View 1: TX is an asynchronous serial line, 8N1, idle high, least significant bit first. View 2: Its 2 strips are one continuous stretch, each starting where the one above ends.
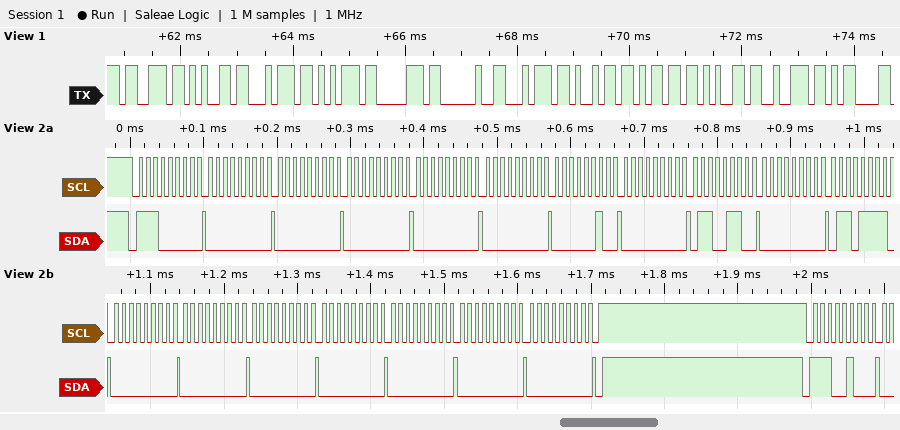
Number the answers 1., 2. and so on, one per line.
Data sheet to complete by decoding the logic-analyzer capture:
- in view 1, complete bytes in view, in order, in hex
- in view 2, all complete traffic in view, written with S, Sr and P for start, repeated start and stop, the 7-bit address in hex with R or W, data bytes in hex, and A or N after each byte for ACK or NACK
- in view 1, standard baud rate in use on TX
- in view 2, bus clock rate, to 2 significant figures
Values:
1. 0x73 0x65 0x74 0x75 0x70 0x20 0x74 0x69 0x6D 0x65 0x72 0x0D
2. S 70W A 00 A 00 A 00 A 00 A 00 A 02 A 00 A 66 A 00 A 6F A 00 A 00 A 00 A 00 A 00 A 00 A 00 A P S 72W A
3. 9600 baud
4. 100 kHz
